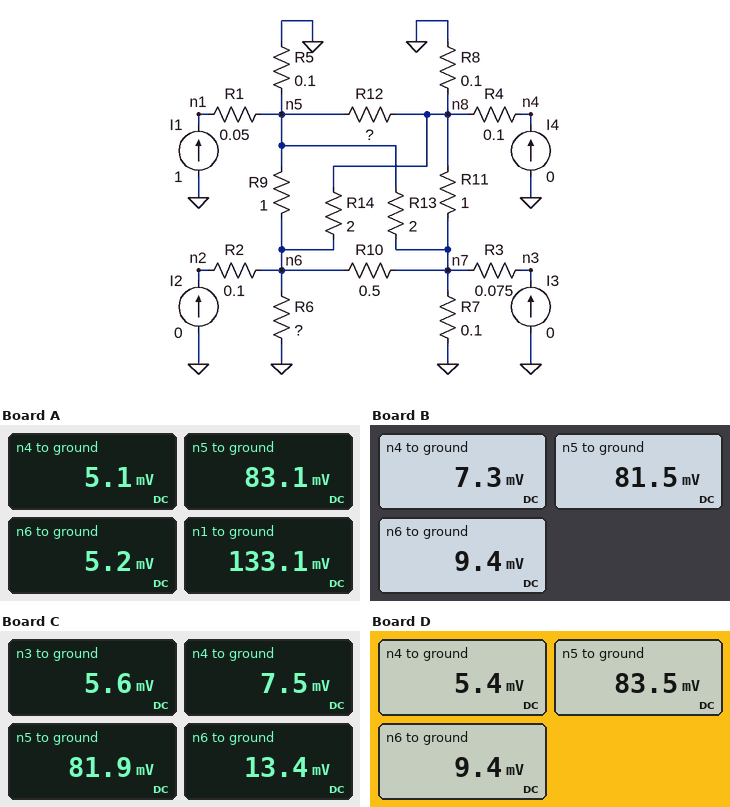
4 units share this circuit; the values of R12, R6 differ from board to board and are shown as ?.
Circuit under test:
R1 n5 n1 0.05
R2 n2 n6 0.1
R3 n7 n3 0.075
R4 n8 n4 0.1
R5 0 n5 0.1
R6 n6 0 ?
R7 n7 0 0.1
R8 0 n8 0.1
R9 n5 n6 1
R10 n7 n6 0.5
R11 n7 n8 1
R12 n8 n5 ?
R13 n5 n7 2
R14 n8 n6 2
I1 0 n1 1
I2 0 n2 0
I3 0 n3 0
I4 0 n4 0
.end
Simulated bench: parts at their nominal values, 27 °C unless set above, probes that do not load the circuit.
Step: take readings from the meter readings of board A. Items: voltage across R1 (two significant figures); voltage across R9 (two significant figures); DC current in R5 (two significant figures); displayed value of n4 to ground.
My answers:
50 mV
78 mV
830 mA
5.1 mV
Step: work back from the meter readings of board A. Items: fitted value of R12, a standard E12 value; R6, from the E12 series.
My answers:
1.5 Ω
0.068 Ω
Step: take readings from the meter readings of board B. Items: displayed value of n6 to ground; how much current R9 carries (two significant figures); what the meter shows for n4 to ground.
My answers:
9.4 mV
72 mA
7.3 mV
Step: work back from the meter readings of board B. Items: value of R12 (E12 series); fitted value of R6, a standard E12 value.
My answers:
1 Ω
0.15 Ω
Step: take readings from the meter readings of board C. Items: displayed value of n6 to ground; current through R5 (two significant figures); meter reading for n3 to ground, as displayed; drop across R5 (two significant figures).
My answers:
13.4 mV
820 mA
5.6 mV
82 mV
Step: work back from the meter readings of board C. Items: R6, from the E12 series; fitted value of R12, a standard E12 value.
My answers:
0.27 Ω
1 Ω
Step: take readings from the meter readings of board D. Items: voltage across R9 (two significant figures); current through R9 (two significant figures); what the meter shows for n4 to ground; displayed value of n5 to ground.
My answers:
74 mV
74 mA
5.4 mV
83.5 mV
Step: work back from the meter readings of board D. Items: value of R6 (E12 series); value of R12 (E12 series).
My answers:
0.15 Ω
1.5 Ω
